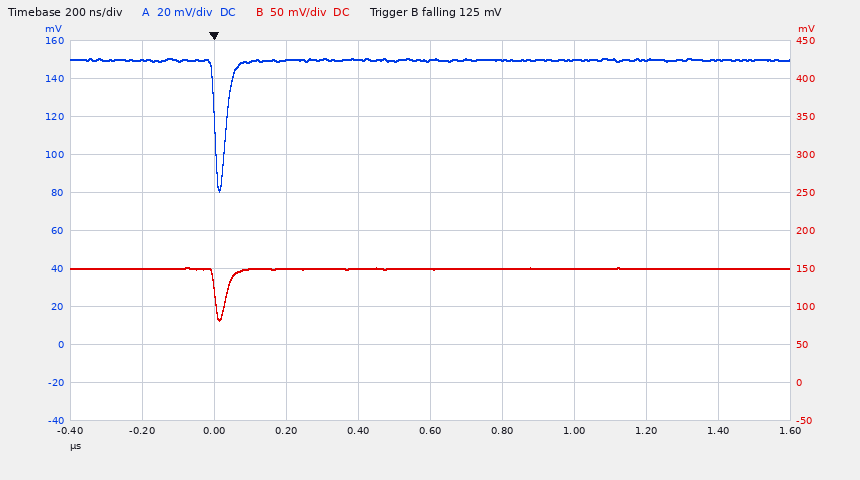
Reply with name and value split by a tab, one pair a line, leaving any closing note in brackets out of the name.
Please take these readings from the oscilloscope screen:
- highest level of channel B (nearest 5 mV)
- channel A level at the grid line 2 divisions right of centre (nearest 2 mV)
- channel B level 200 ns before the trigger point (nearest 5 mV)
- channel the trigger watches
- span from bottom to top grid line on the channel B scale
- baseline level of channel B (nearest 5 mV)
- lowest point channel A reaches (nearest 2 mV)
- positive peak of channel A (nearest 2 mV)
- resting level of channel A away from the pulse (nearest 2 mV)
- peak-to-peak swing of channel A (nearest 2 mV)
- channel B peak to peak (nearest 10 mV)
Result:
highest level of channel B	150 mV
channel A level at the grid line 2 divisions right of centre	150 mV
channel B level 200 ns before the trigger point	150 mV
channel the trigger watches	channel B
span from bottom to top grid line on the channel B scale	500 mV
baseline level of channel B	150 mV
lowest point channel A reaches	80 mV
positive peak of channel A	150 mV
resting level of channel A away from the pulse	150 mV
peak-to-peak swing of channel A	70 mV
channel B peak to peak	70 mV
